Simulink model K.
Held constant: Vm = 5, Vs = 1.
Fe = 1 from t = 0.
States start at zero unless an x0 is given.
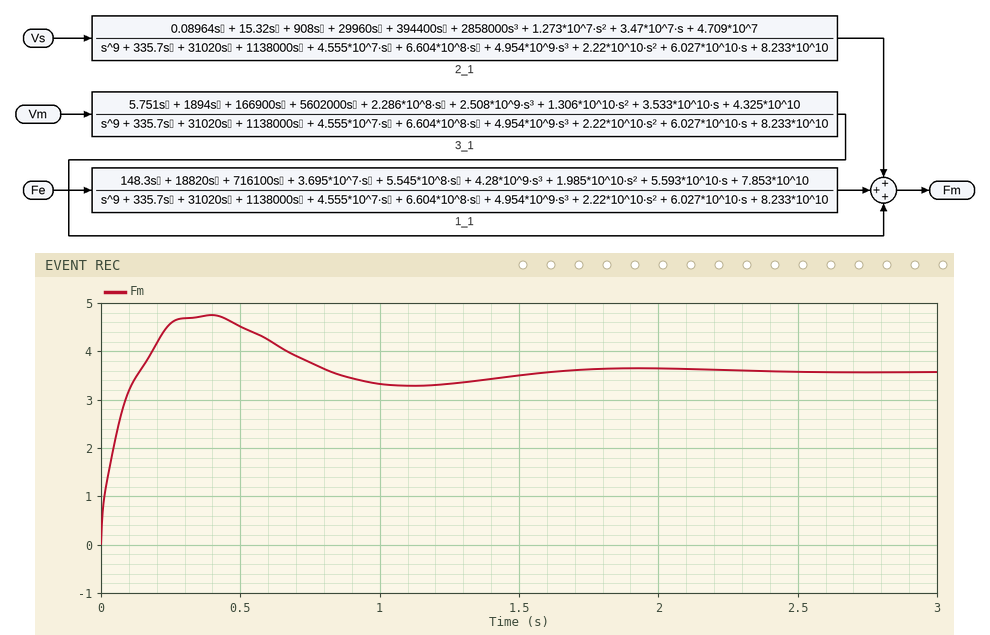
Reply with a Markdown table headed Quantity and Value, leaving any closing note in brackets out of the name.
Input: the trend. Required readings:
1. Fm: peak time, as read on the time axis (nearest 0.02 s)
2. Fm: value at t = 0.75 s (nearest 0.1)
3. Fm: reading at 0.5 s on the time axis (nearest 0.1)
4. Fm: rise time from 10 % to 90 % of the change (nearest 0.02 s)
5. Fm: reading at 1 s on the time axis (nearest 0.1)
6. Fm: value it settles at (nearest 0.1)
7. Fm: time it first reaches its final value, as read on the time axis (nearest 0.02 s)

| Quantity | Value |
|---|---|
| Fm: peak time, as read on the time axis | 0.40 s |
| Fm: value at t = 0.75 s | 3.8 |
| Fm: reading at 0.5 s on the time axis | 4.5 |
| Fm: rise time from 10 % to 90 % of the change | 0.10 s |
| Fm: reading at 1 s on the time axis | 3.3 |
| Fm: value it settles at | 3.6 |
| Fm: time it first reaches its final value, as read on the time axis | 0.14 s |
